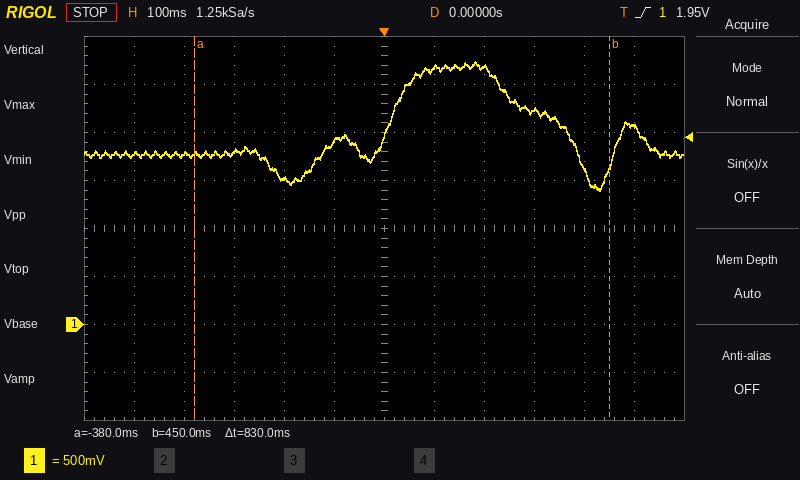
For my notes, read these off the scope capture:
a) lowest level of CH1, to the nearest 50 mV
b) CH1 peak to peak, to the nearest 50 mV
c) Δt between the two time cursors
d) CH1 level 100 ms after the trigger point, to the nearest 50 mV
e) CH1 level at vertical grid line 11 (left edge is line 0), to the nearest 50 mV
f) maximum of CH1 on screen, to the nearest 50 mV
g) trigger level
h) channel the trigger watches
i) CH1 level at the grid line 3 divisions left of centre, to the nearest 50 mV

1.40 V
1.35 V
830 ms
2.65 V
2.05 V
2.75 V
1.95 V
CH1
1.80 V
